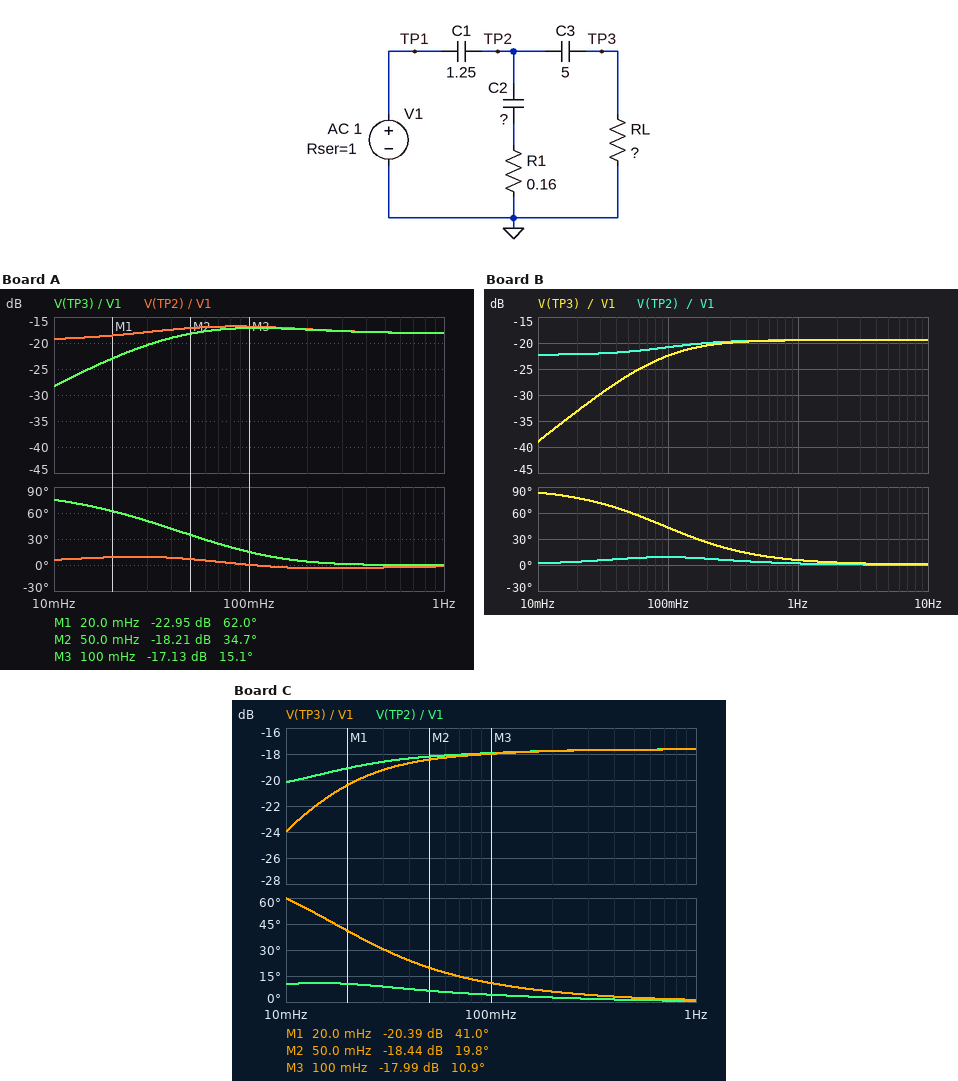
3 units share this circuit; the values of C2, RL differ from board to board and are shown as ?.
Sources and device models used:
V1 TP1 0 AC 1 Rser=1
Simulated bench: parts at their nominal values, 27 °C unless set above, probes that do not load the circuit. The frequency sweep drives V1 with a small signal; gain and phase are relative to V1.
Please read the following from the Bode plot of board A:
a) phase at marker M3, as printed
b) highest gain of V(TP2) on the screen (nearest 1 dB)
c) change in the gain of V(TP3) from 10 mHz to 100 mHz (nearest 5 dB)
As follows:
15.1 deg
-17 dB
10 dB
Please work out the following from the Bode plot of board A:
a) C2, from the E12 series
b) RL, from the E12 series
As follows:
5.6 F
1.2 Ω
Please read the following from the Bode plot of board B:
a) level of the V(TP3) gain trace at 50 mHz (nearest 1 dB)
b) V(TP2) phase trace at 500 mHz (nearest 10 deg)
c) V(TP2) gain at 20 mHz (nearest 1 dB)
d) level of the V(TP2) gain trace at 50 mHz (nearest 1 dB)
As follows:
-26 dB
0 deg
-22 dB
-22 dB
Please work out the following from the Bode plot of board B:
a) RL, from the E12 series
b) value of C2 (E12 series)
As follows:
0.47 Ω
10 F
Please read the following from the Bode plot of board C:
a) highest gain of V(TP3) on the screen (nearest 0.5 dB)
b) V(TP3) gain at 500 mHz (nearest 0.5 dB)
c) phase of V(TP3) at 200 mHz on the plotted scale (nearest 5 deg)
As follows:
-17.5 dB
-17.5 dB
5 deg
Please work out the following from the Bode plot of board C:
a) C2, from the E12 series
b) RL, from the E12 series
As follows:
8.2 F
2.7 Ω
